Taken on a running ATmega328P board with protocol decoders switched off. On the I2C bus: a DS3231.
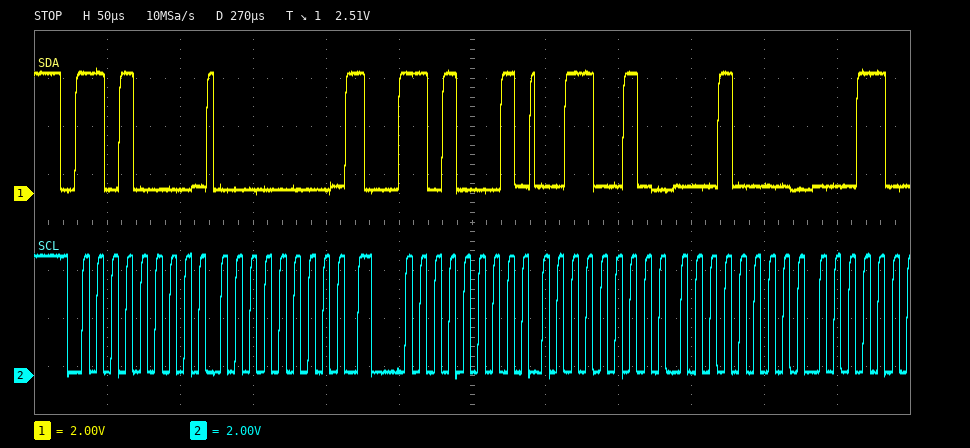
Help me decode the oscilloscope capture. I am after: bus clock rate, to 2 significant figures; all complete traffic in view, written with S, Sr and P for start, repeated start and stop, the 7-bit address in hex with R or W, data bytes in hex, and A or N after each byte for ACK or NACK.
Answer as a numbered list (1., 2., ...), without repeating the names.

1. 100 kHz
2. S 68W A 00 A Sr 68R A 32 A 10 A
